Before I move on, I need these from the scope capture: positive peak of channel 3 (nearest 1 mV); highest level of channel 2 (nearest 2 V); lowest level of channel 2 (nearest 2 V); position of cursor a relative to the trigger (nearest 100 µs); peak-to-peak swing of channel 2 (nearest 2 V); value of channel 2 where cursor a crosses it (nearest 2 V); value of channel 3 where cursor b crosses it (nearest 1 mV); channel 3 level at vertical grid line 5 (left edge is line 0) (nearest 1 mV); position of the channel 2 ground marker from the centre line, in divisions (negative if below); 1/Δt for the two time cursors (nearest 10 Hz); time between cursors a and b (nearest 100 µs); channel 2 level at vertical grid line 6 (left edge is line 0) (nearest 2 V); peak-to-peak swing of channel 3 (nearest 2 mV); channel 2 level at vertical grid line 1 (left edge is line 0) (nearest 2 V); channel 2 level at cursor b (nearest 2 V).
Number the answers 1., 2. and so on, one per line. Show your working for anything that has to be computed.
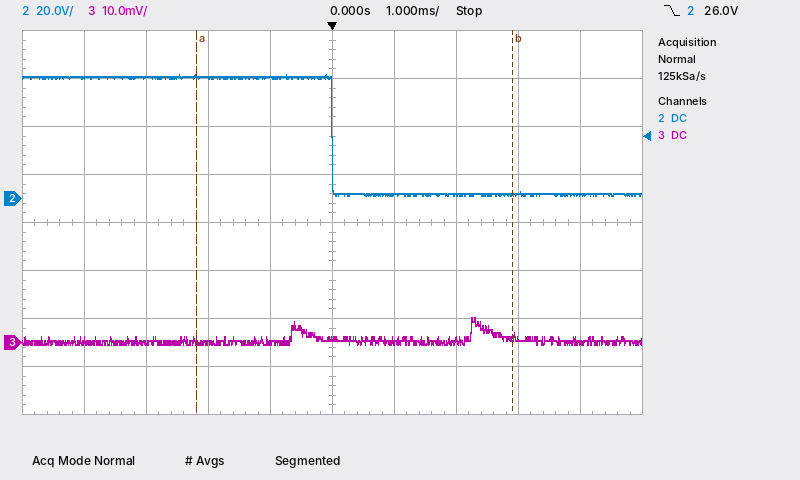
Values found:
1. 5 mV
2. 52 V
3. 2 V
4. -2.2 ms
5. 52 V − (2 V) = 50 V
6. 50 V
7. 1 mV
8. 1 mV
9. +0.5 div
10. 1 / 5.1 ms ≈ 200 Hz
11. 5.1 ms
12. 2 V
13. 6 mV
14. 50 V
15. 2 V
